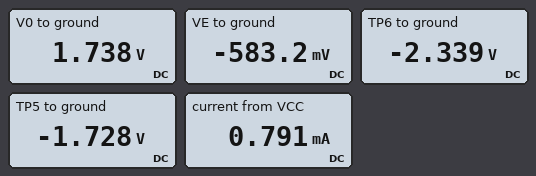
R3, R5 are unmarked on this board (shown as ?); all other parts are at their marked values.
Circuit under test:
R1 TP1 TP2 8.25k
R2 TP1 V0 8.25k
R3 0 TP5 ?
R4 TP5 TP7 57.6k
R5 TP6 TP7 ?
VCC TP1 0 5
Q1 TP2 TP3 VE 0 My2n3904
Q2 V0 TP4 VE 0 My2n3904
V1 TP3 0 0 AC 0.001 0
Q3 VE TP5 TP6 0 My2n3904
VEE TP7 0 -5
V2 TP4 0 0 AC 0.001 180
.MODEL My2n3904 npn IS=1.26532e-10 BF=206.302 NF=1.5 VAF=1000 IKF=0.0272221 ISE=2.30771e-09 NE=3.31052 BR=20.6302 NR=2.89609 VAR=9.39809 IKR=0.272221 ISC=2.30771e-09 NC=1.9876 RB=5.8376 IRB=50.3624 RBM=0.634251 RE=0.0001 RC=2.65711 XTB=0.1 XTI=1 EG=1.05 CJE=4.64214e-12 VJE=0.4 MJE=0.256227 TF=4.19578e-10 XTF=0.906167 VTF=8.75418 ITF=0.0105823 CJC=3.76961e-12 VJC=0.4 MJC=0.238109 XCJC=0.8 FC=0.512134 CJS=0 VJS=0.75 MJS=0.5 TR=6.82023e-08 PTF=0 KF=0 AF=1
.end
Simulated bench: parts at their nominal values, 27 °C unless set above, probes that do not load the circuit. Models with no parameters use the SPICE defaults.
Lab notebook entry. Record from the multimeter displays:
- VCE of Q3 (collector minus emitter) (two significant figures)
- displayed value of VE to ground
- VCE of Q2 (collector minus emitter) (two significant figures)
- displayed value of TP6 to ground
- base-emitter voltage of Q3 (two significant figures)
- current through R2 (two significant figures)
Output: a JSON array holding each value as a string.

["1.8 V", "-583.2 mV", "2.3 V", "-2.339 V", "610 mV", "400 µA"]
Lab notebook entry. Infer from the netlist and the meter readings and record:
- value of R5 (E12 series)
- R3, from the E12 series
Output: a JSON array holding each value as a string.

["3.3 kΩ", "27 kΩ"]
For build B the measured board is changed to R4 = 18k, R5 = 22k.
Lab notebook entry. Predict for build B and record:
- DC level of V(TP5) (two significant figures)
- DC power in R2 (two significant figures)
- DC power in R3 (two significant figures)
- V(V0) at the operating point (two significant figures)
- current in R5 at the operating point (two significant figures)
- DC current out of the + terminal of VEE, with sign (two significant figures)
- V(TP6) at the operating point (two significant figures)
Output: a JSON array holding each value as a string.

["-3.0 V", "8.5 µW", "340 µW", "4.7 V", "67 µA", "-180 µA", "-3.5 V"]
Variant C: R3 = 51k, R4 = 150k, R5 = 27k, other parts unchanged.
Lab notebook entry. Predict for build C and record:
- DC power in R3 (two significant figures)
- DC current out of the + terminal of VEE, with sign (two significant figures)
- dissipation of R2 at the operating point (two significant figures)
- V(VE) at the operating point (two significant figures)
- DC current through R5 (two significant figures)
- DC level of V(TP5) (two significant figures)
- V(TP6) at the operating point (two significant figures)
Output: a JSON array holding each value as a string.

["35 µW", "-140 µA", "26 µW", "-510 mV", "120 µA", "-1.3 V", "-1.9 V"]
